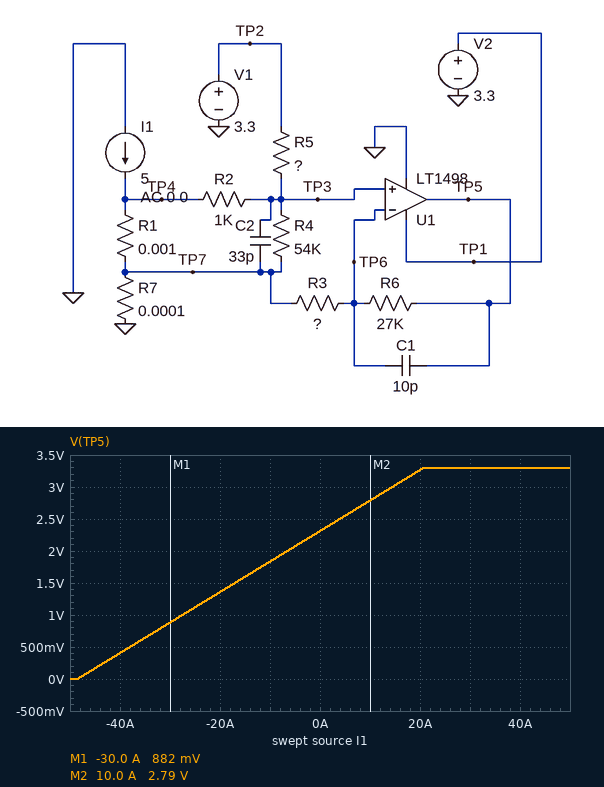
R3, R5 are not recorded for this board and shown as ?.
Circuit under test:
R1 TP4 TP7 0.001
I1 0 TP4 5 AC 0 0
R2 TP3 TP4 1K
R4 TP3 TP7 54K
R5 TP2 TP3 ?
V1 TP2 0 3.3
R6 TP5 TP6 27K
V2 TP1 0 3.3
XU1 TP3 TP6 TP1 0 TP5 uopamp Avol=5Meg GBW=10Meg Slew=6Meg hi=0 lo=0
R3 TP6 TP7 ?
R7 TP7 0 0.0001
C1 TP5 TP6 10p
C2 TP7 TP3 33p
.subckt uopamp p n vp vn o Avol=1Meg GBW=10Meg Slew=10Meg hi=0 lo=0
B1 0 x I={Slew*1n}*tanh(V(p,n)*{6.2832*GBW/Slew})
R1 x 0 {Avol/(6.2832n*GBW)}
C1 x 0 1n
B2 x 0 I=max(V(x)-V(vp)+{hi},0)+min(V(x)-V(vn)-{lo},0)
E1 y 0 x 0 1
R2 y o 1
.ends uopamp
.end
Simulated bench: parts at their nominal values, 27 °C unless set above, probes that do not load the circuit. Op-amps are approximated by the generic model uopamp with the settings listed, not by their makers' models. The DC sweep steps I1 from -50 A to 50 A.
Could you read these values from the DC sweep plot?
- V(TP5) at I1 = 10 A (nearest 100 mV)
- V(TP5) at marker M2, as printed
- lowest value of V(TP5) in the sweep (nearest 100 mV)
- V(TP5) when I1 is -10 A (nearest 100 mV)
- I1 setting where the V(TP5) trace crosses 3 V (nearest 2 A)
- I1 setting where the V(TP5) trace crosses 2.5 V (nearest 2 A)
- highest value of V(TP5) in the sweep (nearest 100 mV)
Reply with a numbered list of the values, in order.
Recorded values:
1. 2.8 V
2. 2.79 V
3. 0 V
4. 1.8 V
5. 14 A
6. 4 A
7. 3.3 V
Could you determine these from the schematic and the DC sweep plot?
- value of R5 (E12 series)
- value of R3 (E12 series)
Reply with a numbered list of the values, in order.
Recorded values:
1. 68 kΩ
2. 560 Ω
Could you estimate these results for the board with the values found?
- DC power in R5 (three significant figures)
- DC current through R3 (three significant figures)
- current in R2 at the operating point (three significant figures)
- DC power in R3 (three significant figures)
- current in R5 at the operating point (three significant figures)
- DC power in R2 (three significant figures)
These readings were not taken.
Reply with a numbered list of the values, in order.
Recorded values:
1. 155 µW
2. 92.5 µA
3. 46.8 µA
4. 4.79 µW
5. 47.8 µA
6. 2.19 µW
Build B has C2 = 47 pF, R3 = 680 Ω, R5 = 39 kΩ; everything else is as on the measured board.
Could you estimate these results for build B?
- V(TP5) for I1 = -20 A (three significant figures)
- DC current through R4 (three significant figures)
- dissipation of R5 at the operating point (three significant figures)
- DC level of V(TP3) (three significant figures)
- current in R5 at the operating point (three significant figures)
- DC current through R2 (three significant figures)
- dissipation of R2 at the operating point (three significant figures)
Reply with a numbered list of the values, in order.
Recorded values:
1. 2.52 V
2. 1.59 µA
3. 265 µW
4. 86.3 mV
5. 82.4 µA
6. 80.8 µA
7. 6.53 µW
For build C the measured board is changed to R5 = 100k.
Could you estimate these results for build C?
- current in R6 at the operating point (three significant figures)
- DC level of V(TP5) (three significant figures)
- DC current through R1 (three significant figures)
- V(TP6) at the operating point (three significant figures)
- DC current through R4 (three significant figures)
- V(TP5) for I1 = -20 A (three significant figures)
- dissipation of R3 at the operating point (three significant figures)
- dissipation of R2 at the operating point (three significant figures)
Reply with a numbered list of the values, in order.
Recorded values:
1. 66.0 µA
2. 1.82 V
3. 5.00 A
4. 37.4 mV
5. 684 nA
6. 621 mV
7. 2.44 µW
8. 1.02 µW
